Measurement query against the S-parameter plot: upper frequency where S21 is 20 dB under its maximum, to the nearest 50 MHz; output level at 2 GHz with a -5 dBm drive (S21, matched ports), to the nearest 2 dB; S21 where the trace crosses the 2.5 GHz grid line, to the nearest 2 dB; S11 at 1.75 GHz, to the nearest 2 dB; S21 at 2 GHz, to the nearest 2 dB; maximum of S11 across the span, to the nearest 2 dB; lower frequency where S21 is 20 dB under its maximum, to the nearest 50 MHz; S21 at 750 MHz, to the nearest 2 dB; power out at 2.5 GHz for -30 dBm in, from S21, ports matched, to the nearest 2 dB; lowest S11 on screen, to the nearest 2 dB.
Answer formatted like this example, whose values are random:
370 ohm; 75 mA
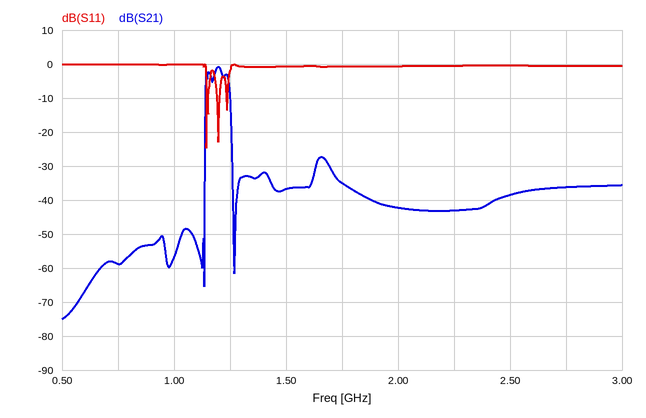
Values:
1.25 GHz; -48 dBm; -38 dB; 0 dB; -42 dB; 0 dB; 1.15 GHz; -58 dB; -68 dBm; -24 dB
